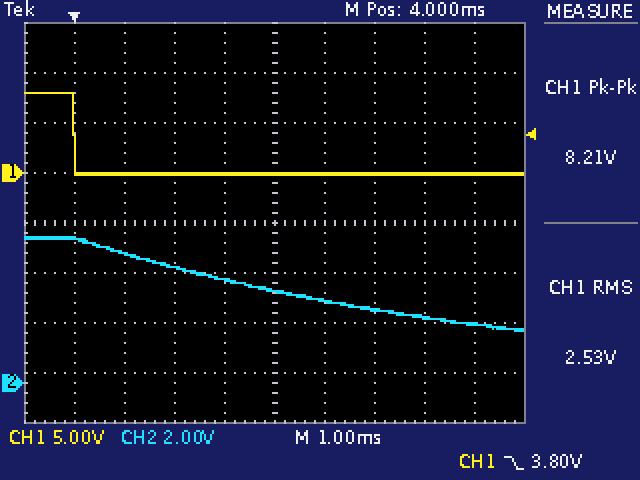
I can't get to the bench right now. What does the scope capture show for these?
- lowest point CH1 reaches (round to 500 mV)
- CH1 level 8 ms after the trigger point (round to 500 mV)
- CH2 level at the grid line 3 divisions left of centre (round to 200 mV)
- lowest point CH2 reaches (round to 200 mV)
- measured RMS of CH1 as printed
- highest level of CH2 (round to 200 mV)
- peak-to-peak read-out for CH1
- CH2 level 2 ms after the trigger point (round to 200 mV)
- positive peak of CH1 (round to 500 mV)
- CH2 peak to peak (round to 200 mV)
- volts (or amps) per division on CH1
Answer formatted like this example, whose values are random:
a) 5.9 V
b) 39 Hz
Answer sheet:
a) 0.0 V
b) 0.0 V
c) 5.2 V
d) 2.0 V
e) 2.53 V
f) 5.8 V
g) 8.21 V
h) 4.6 V
i) 8.0 V
j) 3.8 V
k) 5 V
